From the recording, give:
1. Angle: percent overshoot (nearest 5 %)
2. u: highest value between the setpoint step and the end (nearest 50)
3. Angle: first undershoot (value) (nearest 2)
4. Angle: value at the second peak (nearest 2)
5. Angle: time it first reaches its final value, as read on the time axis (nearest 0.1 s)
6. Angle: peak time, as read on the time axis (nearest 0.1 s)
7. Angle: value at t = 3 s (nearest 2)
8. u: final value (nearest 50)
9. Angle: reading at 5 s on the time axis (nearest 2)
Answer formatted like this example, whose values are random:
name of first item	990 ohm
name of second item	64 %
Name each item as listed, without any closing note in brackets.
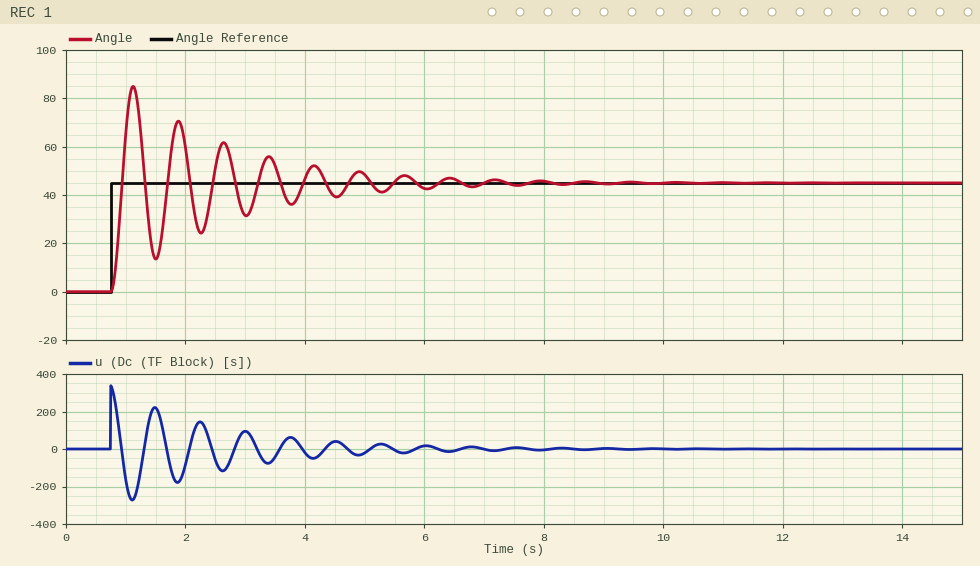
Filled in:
Angle: percent overshoot	90 %
u: highest value between the setpoint step and the end	350
Angle: first undershoot (value)	14
Angle: value at the second peak	70
Angle: time it first reaches its final value, as read on the time axis	0.9 s
Angle: peak time, as read on the time axis	1.1 s
Angle: value at t = 3 s	32
u: final value	0
Angle: reading at 5 s on the time axis	48
